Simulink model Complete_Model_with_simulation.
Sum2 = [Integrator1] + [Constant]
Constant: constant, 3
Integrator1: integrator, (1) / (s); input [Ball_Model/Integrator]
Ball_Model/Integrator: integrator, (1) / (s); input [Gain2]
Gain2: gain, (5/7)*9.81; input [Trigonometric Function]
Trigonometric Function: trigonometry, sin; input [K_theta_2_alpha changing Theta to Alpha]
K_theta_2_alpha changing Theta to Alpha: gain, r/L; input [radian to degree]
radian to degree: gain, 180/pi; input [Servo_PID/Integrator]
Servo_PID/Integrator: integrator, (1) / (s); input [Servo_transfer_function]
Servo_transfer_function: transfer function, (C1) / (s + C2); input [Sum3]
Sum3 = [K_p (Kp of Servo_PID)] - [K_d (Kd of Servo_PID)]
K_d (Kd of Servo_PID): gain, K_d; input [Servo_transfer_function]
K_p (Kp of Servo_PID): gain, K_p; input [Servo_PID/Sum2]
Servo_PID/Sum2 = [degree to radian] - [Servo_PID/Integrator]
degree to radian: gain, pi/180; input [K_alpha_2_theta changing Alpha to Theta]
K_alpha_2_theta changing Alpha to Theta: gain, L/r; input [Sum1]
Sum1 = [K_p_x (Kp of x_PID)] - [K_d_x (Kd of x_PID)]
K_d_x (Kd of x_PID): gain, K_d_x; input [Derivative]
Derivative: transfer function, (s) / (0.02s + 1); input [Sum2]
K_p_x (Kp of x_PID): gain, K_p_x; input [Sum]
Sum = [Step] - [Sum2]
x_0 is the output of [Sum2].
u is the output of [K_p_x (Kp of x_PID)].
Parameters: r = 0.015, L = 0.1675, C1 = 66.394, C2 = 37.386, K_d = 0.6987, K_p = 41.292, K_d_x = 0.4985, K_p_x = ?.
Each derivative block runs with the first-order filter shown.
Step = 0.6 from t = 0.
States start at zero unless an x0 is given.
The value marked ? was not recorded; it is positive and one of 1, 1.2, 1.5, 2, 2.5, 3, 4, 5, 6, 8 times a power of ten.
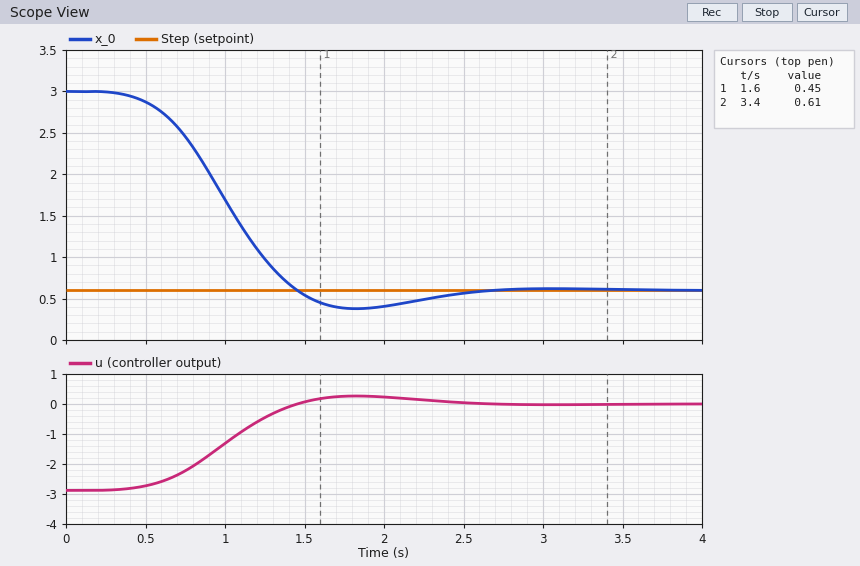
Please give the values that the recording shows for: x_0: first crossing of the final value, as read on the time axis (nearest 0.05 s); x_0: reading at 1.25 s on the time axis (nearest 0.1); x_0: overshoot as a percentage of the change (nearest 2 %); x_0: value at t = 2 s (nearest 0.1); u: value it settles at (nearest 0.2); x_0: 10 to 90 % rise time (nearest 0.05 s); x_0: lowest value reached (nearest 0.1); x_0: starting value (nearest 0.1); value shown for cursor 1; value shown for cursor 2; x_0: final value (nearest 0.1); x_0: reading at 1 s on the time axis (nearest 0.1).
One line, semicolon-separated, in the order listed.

1.45 s; 1.0; 10 %; 0.4; 0.0; 0.70 s; 0.4; 3.0; 0.45; 0.61; 0.6; 1.7
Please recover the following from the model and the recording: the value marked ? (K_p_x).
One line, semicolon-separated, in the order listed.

1.2
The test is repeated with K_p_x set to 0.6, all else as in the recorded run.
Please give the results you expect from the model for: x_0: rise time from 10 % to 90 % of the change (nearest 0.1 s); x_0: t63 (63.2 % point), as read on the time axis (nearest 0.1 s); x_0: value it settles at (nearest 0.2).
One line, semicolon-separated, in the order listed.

1.3 s; 1.1 s; 0.6
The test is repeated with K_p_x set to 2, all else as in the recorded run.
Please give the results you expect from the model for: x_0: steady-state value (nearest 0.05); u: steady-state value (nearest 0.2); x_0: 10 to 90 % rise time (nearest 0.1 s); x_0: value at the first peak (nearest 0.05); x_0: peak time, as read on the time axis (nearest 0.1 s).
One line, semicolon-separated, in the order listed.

3.75; -6.2; 0.4 s; 3.90; 1.1 s
